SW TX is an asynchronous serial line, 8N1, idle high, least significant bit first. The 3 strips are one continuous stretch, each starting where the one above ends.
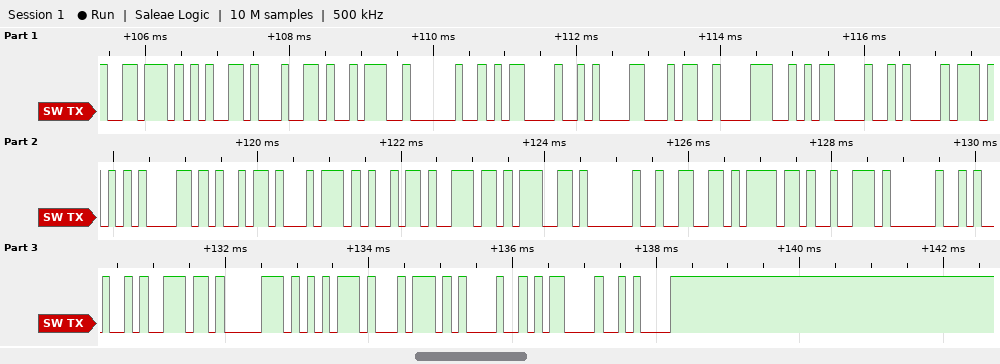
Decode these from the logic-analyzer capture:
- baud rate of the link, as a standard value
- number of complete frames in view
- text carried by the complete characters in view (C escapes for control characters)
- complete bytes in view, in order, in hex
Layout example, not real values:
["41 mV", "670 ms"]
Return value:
["9600 baud", "31", "\"ved: \\r\\n48\\r\\nWaiting for Input!\\r\\n\"", "76 65 64 3A 20 0D 0A 34 38 0D 0A 57 61 69 74 69 6E 67 20 66 6F 72 20 49 6E 70 75 74 21 0D 0A"]
